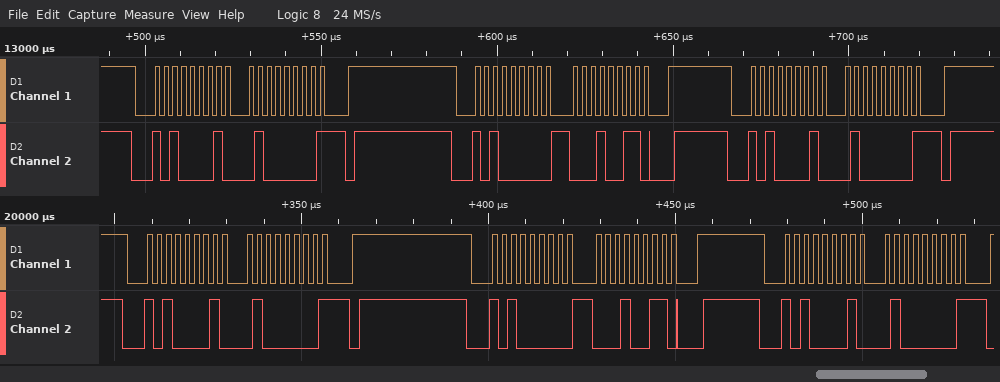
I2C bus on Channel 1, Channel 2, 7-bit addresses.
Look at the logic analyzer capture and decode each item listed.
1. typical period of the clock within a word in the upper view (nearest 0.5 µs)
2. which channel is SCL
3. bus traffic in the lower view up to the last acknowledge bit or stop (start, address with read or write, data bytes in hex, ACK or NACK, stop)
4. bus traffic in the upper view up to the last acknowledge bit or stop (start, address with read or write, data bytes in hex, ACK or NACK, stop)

2.5 µs
Channel 1
start, address 50 read ACK, 40 NACK, stop, start, address 50 write ACK, 13 ACK, stop, start, address 50 read ACK, 40 NACK
start, address 50 read ACK, 40 NACK, stop, start, address 50 write ACK, 13 ACK, stop, start, address 50 read ACK, 40 NACK, stop
